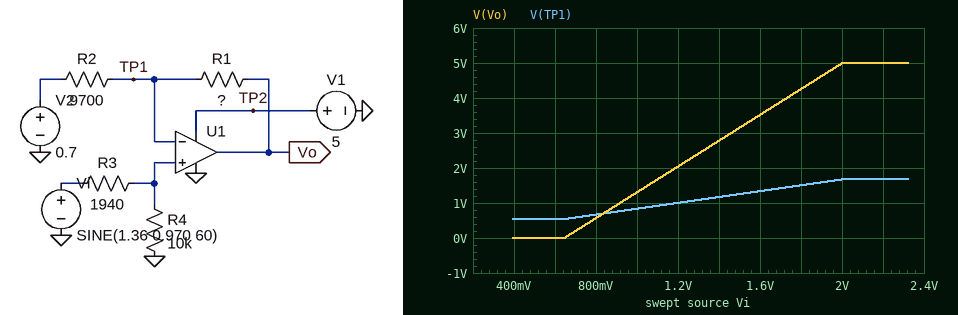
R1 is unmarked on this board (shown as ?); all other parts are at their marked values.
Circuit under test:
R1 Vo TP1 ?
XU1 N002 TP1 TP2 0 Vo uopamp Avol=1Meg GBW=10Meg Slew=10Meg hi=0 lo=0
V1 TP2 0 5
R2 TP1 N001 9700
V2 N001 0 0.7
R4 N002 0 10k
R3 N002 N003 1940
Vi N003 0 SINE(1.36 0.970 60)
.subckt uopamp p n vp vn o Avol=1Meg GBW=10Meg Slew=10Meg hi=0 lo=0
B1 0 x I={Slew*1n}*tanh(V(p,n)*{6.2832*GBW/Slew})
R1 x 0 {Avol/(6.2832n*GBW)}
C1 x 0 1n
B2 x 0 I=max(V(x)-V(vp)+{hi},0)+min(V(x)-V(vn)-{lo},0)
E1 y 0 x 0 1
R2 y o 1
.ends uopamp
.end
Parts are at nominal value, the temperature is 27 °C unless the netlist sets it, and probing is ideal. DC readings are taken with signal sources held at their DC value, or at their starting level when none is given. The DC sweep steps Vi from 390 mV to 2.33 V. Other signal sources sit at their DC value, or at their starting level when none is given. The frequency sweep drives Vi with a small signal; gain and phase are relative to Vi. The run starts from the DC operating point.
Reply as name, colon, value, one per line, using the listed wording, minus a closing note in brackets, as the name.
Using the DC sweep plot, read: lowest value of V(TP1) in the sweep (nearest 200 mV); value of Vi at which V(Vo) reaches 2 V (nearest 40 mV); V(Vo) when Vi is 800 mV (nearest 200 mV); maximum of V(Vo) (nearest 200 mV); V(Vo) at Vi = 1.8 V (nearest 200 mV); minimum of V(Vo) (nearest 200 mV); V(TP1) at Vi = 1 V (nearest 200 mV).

lowest value of V(TP1) in the sweep: 600 mV
value of Vi at which V(Vo) reaches 2 V: 1.20 V
V(Vo) when Vi is 800 mV: 600 mV
maximum of V(Vo): 5.0 V
V(Vo) at Vi = 1.8 V: 4.2 V
minimum of V(Vo): 0 V
V(TP1) at Vi = 1 V: 800 mV
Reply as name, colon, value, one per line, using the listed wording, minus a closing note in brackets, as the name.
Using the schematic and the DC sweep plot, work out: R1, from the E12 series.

R1, from the E12 series: 33 kΩ
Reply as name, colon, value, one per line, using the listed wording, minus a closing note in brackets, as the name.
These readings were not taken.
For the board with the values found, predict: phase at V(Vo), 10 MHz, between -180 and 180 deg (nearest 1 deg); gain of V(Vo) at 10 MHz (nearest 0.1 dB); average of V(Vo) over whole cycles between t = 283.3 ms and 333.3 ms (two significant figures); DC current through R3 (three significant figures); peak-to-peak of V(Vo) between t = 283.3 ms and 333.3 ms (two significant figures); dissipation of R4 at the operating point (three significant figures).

phase at V(Vo), 10 MHz, between -180 and 180 deg: -77 deg
gain of V(Vo) at 10 MHz: -1.8 dB
average of V(Vo) over whole cycles between t = 283.3 ms and 333.3 ms: 2.6 V
DC current through R3: 114 µA
peak-to-peak of V(Vo) between t = 283.3 ms and 333.3 ms: 5.0 V
dissipation of R4 at the operating point: 130 µW
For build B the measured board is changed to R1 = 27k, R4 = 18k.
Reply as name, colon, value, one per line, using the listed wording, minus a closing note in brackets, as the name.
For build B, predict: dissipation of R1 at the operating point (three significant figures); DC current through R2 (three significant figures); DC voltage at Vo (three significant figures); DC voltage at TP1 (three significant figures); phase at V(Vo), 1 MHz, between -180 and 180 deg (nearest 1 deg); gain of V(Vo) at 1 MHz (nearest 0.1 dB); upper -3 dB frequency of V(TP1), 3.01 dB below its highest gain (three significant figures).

dissipation of R1 at the operating point: 79.9 µW
DC current through R2: 54.4 µA
DC voltage at Vo: 2.70 V
DC voltage at TP1: 1.23 V
phase at V(Vo), 1 MHz, between -180 and 180 deg: -21 deg
gain of V(Vo) at 1 MHz: 10.1 dB
upper -3 dB frequency of V(TP1), 3.01 dB below its highest gain: 2.64 MHz
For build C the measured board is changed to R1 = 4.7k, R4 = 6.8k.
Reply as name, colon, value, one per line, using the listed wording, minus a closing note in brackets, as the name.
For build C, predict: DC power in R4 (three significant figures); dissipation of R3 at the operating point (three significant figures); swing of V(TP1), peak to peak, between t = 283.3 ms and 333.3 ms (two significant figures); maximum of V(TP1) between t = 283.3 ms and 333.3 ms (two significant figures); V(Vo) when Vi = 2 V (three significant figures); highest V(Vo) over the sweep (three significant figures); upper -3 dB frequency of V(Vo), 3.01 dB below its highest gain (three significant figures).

DC power in R4: 165 µW
dissipation of R3 at the operating point: 47.0 µW
swing of V(TP1), peak to peak, between t = 283.3 ms and 333.3 ms: 1.5 V
maximum of V(TP1) between t = 283.3 ms and 333.3 ms: 1.8 V
V(Vo) when Vi = 2 V: 1.97 V
highest V(Vo) over the sweep: 2.35 V
upper -3 dB frequency of V(Vo), 3.01 dB below its highest gain: 6.74 MHz
